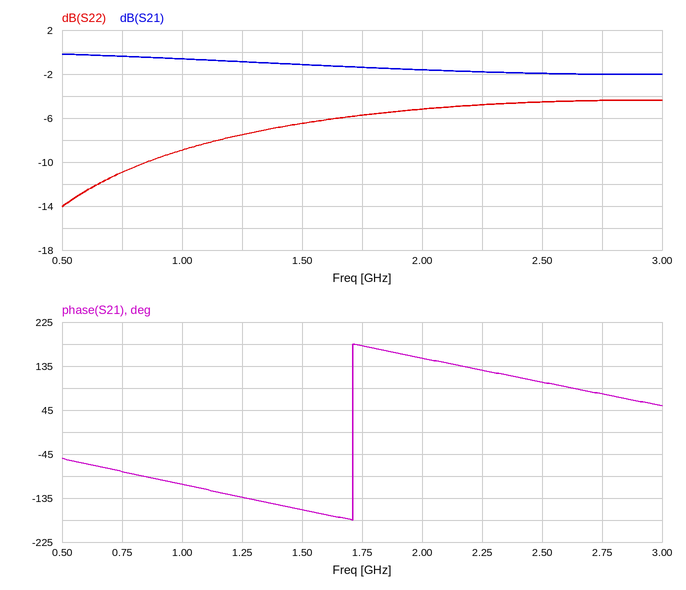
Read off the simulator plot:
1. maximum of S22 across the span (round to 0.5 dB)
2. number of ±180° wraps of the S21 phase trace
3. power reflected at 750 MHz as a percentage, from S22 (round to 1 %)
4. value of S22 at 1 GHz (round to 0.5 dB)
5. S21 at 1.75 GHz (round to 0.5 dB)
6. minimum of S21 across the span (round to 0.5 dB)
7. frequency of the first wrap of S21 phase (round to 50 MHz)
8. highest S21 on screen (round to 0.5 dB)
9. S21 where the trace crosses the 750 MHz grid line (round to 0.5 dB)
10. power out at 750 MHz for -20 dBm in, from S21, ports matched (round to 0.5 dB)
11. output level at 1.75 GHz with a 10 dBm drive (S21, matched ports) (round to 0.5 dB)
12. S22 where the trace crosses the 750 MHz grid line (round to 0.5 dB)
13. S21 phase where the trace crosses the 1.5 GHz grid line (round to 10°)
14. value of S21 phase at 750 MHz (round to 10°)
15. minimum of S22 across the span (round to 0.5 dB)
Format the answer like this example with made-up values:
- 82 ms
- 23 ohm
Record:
- -4.5 dB
- 1
- 8 %
- -9.0 dB
- -1.5 dB
- -2.0 dB
- 1.70 GHz
- 0.0 dB
- -0.5 dB
- -20.5 dBm
- 8.5 dBm
- -11.0 dB
- -160°
- -80°
- -14.0 dB
